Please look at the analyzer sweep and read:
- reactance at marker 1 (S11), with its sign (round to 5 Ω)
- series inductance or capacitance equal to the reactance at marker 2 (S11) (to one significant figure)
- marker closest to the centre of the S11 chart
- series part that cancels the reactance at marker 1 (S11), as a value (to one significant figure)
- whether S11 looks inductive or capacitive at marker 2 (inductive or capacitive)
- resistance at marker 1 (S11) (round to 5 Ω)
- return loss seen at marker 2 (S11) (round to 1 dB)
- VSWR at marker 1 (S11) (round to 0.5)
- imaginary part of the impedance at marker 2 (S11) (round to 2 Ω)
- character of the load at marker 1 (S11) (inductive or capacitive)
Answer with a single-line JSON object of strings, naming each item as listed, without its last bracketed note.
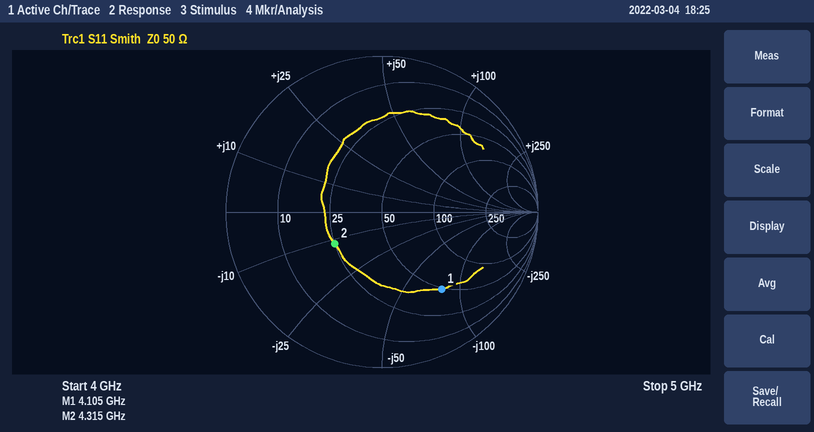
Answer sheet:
{"reactance at marker 1 (S11), with its sign": "-80 Ω", "series inductance or capacitance equal to the reactance at marker 2 (S11)": "3 pF", "marker closest to the centre of the S11 chart": "marker 2", "series part that cancels the reactance at marker 1 (S11), as a value": "3 nH", "whether S11 looks inductive or capacitive at marker 2": "capacitive", "resistance at marker 1 (S11)": "50 Ω", "return loss seen at marker 2 (S11)": "9 dB", "VSWR at marker 1 (S11)": "4.5", "imaginary part of the impedance at marker 2 (S11)": "-12 Ω", "character of the load at marker 1 (S11)": "capacitive"}
